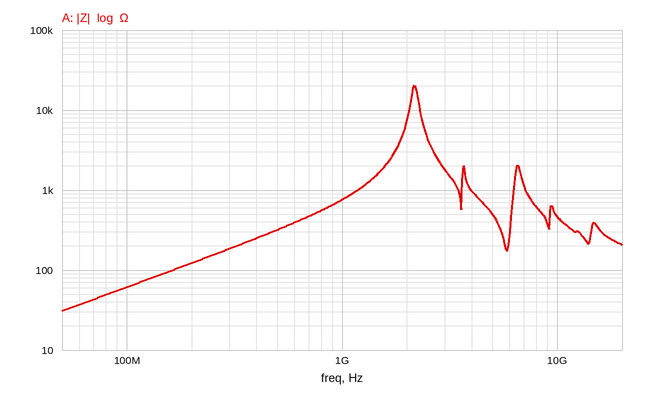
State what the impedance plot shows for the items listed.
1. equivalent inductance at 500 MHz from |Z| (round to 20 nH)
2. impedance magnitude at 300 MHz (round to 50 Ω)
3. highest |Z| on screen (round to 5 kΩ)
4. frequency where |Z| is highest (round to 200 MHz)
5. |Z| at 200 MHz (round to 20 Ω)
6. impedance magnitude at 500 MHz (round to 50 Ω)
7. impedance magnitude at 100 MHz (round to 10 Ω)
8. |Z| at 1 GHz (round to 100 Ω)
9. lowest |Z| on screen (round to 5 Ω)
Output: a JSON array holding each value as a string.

["100 nH", "200 Ω", "20 kΩ", "2.2 GHz", "120 Ω", "300 Ω", "60 Ω", "800 Ω", "30 Ω"]
